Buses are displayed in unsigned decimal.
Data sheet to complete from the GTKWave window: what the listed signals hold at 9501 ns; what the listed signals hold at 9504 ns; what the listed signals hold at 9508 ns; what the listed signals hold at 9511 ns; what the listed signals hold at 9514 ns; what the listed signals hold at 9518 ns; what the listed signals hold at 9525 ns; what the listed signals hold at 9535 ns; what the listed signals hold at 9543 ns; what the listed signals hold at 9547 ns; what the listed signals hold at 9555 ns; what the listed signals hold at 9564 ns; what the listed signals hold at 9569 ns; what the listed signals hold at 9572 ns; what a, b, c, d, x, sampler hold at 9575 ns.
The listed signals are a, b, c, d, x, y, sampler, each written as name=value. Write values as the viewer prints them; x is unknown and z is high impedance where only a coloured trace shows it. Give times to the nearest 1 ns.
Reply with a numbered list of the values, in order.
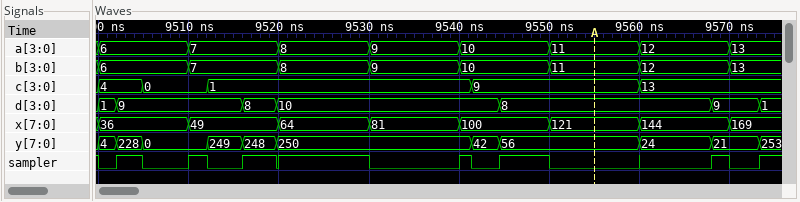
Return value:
1. a=6, b=6, c=4, d=1, x=36, y=4, sampler=0
2. a=6, b=6, c=4, d=9, x=36, y=228, sampler=1
3. a=6, b=6, c=0, d=9, x=36, y=0, sampler=0
4. a=7, b=7, c=0, d=9, x=49, y=0, sampler=1
5. a=7, b=7, c=1, d=9, x=49, y=249, sampler=0
6. a=7, b=7, c=1, d=8, x=49, y=248, sampler=1
7. a=8, b=8, c=1, d=10, x=64, y=250, sampler=1
8. a=9, b=9, c=1, d=10, x=81, y=250, sampler=0
9. a=10, b=10, c=9, d=10, x=100, y=42, sampler=0
10. a=10, b=10, c=9, d=8, x=100, y=56, sampler=1
11. a=11, b=11, c=9, d=8, x=121, y=56, sampler=0
12. a=12, b=12, c=13, d=8, x=144, y=24, sampler=0
13. a=12, b=12, c=13, d=9, x=144, y=21, sampler=1
14. a=13, b=13, c=13, d=9, x=169, y=21, sampler=0
15. a=13, b=13, c=13, d=1, x=169, sampler=1
